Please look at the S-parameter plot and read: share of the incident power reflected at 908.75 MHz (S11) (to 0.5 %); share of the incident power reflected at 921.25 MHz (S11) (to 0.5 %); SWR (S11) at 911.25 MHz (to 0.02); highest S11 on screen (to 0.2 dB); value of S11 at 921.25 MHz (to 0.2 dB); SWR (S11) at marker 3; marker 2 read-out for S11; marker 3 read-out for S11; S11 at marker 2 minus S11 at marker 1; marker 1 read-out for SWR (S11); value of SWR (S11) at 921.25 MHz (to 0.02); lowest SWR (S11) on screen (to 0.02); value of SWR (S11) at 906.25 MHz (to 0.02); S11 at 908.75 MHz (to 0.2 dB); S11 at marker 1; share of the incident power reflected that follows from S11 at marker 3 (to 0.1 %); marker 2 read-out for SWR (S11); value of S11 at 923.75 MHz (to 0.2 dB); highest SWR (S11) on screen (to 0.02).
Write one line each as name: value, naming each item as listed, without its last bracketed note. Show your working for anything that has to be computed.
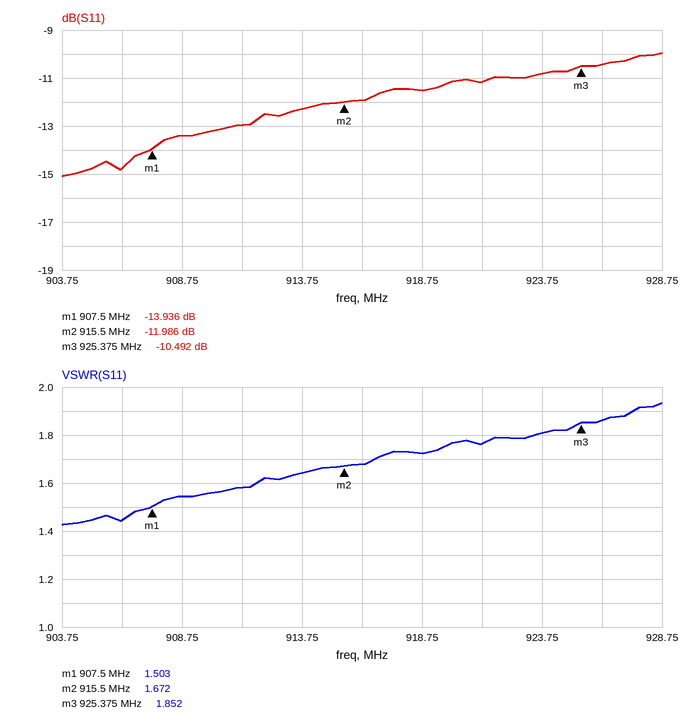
share of the incident power reflected at 908.75 MHz (S11): 10^(-13.4/10) ≈ 4.57 %, so 4.5 % to the nearest 0.5 %
share of the incident power reflected at 921.25 MHz (S11): 10^(-11.2/10) ≈ 7.59 %, so 7.5 % to the nearest 0.5 %
SWR (S11) at 911.25 MHz: 1.58
highest S11 on screen: -10.0 dB
value of S11 at 921.25 MHz: -11.2 dB
SWR (S11) at marker 3: 1.852
marker 2 read-out for S11: -11.986 dB
marker 3 read-out for S11: -10.492 dB
S11 at marker 2 minus S11 at marker 1: -11.986 − (-13.936) = 1.950 dB
marker 1 read-out for SWR: 1.503
value of SWR (S11) at 921.25 MHz: 1.76
lowest SWR (S11) on screen: 1.42
value of SWR (S11) at 906.25 MHz: 1.44
S11 at 908.75 MHz: -13.4 dB
S11 at marker 1: -13.936 dB
share of the incident power reflected that follows from S11 at marker 3: 10^(-10.492/10) ≈ 8.9 %
marker 2 read-out for SWR: 1.672
value of S11 at 923.75 MHz: -10.8 dB
highest SWR (S11) on screen: 1.94
